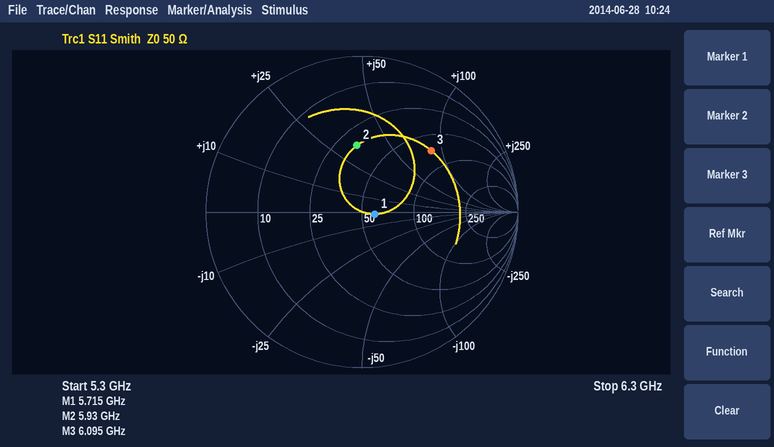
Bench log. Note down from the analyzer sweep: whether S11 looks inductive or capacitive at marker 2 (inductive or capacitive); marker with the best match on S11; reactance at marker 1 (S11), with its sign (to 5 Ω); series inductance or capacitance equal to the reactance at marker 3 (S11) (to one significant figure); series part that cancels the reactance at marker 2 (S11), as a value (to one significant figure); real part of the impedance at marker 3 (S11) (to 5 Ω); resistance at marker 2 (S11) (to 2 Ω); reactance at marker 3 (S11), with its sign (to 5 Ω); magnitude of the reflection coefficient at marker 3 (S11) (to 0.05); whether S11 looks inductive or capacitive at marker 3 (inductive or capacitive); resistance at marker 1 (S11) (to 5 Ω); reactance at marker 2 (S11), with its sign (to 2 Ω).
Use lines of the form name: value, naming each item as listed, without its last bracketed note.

whether S11 looks inductive or capacitive at marker 2: inductive
marker with the best match on S11: marker 1
reactance at marker 1 (S11), with its sign: 0 Ω
series inductance or capacitance equal to the reactance at marker 3 (S11): 2 nH
series part that cancels the reactance at marker 2 (S11), as a value: 800 fF
real part of the impedance at marker 3 (S11): 70 Ω
resistance at marker 2 (S11): 32 Ω
reactance at marker 3 (S11), with its sign: +85 Ω
magnitude of the reflection coefficient at marker 3 (S11): 0.60
whether S11 looks inductive or capacitive at marker 3: inductive
resistance at marker 1 (S11): 60 Ω
reactance at marker 2 (S11), with its sign: +34 Ω
